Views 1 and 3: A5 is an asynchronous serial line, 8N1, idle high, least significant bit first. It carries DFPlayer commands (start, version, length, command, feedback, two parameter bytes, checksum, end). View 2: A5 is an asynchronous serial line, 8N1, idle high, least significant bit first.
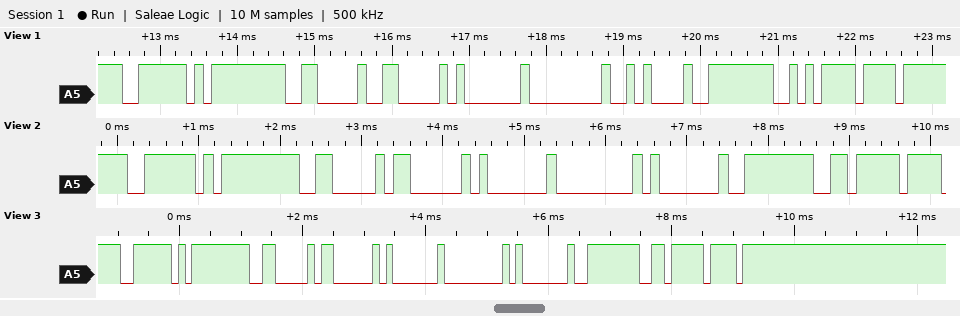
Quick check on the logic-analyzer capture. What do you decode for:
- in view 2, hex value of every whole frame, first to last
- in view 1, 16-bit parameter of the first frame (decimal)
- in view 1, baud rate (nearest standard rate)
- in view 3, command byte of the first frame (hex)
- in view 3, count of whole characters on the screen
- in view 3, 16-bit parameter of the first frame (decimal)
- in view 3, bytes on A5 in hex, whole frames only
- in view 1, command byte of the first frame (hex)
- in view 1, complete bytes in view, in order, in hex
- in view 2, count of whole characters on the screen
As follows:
0x7E 0xFF 0x06 0x03 0x01 0x00 0x01 0xFE 0xF6
10
9600 baud
0x03
10
1
7E FF 06 03 01 00 01 FE F6 EF
0x06
7E FF 06 06 01 00 0A FE EA EF
9
